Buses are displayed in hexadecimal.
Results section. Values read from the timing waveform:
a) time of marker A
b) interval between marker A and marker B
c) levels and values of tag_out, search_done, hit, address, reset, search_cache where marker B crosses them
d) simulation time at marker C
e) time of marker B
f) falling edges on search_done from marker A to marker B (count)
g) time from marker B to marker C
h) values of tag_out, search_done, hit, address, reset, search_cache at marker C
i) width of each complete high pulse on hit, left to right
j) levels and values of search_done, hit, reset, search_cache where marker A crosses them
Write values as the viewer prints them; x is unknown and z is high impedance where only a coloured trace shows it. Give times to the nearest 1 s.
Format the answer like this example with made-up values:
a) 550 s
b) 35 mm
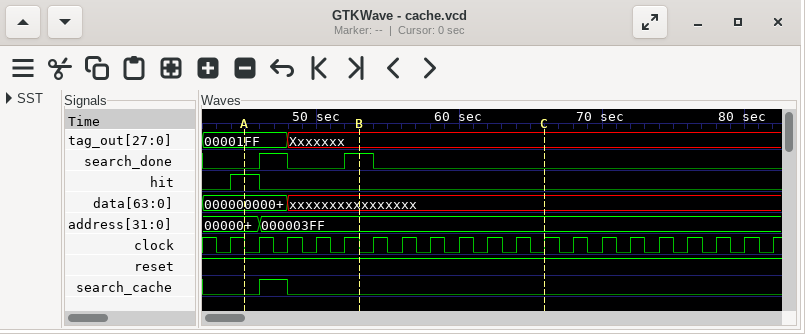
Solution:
a) 45 s
b) 8 s
c) tag_out=Xxxxxxx, search_done=1, hit=0, address=000003FF, reset=1, search_cache=0
d) 66 s
e) 53 s
f) 1
g) 13 s
h) tag_out=Xxxxxxx, search_done=0, hit=0, address=000003FF, reset=1, search_cache=0
i) 2 s
j) search_done=0, hit=1, reset=1, search_cache=0
